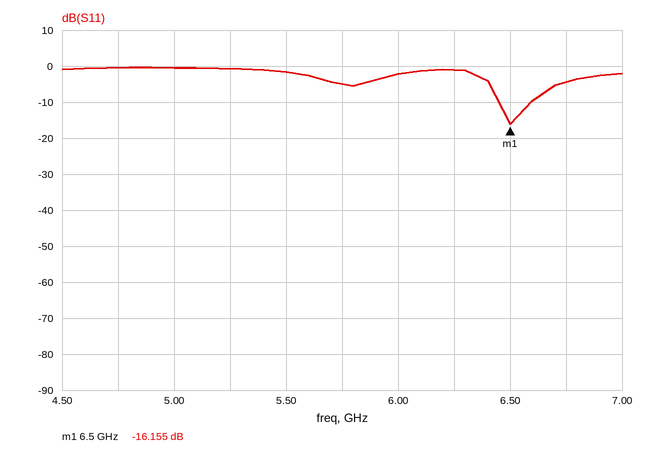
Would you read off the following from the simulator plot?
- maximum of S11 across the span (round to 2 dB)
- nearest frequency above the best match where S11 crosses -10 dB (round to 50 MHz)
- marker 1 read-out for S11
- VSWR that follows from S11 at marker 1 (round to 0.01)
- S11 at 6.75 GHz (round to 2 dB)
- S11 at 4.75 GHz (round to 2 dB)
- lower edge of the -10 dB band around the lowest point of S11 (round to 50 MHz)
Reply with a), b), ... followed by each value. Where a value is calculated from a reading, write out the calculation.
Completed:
a) 0 dB
b) 6.60 GHz
c) -16.155 dB
d) (1 + 0.1557)/(1 − 0.1557) ≈ 1.37
e) -4 dB
f) 0 dB
g) 6.45 GHz
